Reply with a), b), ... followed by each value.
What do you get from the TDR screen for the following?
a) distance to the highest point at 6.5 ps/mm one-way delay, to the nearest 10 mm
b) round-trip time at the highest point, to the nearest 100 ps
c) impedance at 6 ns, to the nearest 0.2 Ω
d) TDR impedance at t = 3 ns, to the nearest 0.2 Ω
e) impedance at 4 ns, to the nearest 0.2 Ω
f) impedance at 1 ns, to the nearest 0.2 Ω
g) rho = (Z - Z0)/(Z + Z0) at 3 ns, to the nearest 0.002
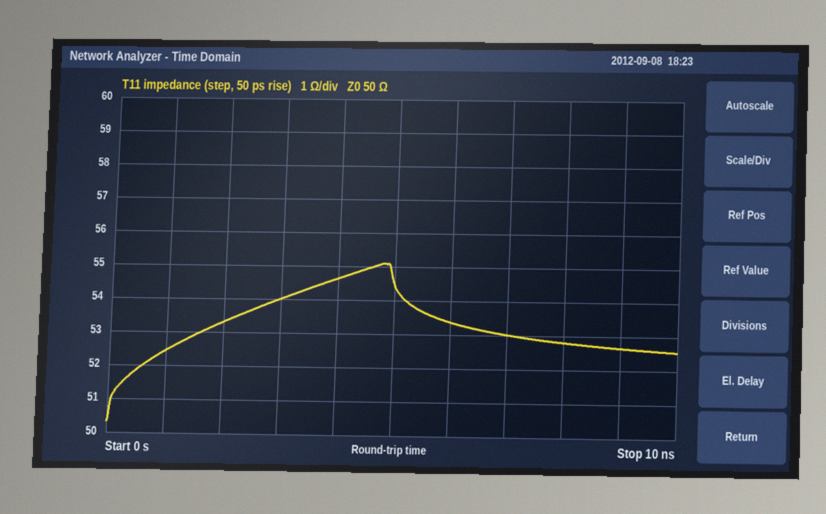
a) 370 mm
b) 4.8 ns
c) 53.4 Ω
d) 54.0 Ω
e) 54.6 Ω
f) 52.4 Ω
g) +0.038
